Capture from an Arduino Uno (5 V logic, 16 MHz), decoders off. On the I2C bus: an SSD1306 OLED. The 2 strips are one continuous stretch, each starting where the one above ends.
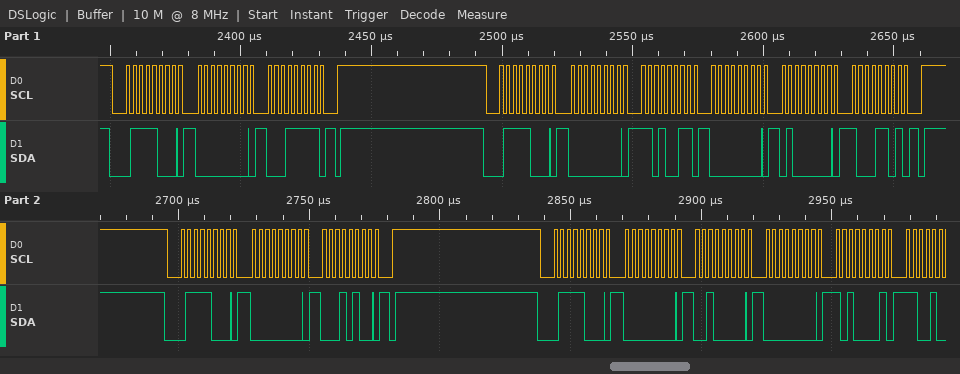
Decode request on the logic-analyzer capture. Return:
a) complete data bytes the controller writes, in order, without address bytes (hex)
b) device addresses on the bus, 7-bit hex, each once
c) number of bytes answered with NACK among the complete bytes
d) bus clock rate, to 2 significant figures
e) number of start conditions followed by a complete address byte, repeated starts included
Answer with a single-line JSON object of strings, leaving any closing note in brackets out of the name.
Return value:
{"complete data bytes the controller writes, in order, without address bytes": "00 1F 00 D3 00 40 8D 00 14 00 20 00 A1", "device addresses on the bus, 7-bit hex, each once": "0x3C", "number of bytes answered with NACK among the complete bytes": "0", "bus clock rate, to 2 significant figures": "400 kHz", "number of start conditions followed by a complete address byte, repeated starts included": "4"}
